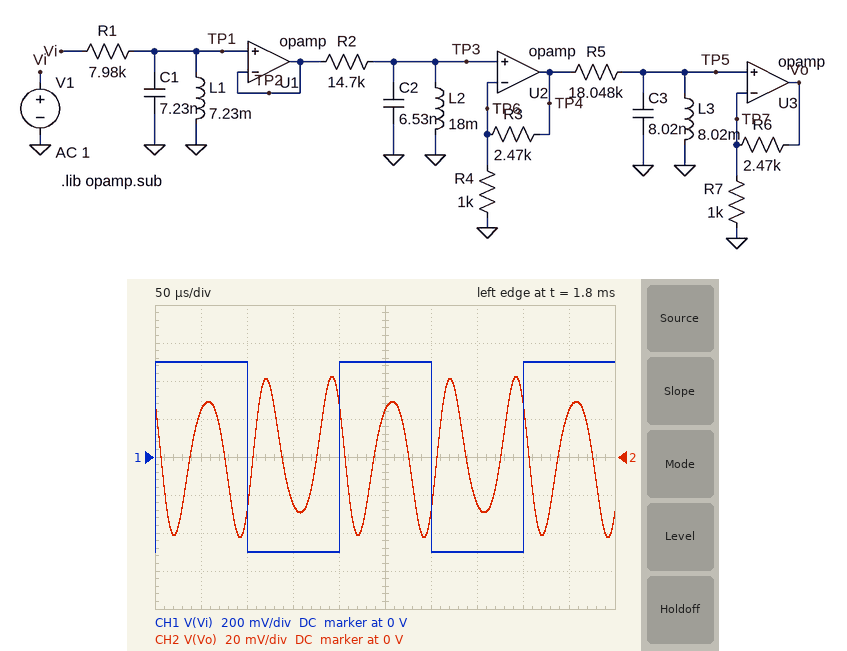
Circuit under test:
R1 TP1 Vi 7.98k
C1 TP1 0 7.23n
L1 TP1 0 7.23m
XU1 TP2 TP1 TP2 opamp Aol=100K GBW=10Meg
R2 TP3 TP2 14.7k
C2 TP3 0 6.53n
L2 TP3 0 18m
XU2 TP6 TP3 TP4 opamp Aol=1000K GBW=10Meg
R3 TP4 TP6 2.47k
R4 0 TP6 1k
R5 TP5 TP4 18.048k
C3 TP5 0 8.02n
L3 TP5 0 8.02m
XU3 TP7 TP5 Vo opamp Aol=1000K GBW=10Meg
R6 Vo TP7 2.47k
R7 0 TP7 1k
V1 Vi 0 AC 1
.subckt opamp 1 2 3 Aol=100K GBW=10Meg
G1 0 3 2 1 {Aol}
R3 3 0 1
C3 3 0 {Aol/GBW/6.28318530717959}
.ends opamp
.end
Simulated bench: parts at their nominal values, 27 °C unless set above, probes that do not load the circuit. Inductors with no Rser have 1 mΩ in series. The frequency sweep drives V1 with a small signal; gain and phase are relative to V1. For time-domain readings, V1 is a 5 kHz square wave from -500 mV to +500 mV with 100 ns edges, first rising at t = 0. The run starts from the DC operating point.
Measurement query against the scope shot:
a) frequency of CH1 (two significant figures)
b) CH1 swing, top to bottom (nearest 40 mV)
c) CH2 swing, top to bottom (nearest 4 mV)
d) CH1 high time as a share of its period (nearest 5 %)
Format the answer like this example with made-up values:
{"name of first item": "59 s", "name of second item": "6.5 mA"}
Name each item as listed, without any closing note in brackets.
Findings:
{"frequency of CH1": "5.0 kHz", "CH1 swing, top to bottom": "1.00 V", "CH2 swing, top to bottom": "84 mV", "CH1 high time as a share of its period": "50 %"}
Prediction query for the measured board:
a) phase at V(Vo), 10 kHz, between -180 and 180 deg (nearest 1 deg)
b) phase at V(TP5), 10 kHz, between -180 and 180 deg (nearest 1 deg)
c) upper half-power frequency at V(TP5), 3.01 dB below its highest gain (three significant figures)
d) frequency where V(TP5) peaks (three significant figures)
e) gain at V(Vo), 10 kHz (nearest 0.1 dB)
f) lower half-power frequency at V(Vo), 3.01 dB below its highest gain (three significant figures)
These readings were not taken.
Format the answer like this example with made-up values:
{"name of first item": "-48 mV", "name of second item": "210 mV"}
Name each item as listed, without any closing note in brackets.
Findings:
{"phase at V(Vo), 10 kHz, between -180 and 180 deg": "-105 deg", "phase at V(TP5), 10 kHz, between -180 and 180 deg": "-105 deg", "upper half-power frequency at V(TP5), 3.01 dB below its highest gain": "20.6 kHz", "frequency where V(TP5) peaks": "19.9 kHz", "gain at V(Vo), 10 kHz": "-46.8 dB", "lower half-power frequency at V(Vo), 3.01 dB below its highest gain": "19.4 kHz"}
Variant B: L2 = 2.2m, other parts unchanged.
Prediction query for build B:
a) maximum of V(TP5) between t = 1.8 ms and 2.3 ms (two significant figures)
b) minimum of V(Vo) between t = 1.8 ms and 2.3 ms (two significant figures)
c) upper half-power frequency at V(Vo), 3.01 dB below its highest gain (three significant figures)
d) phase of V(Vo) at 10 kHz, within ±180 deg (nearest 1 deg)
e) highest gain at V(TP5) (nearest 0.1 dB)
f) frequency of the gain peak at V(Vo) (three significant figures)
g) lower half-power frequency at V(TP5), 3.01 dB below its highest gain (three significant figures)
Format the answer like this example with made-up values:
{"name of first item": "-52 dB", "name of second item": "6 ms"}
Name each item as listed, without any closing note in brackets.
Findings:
{"maximum of V(TP5) between t = 1.8 ms and 2.3 ms": "1.1 mV", "minimum of V(Vo) between t = 1.8 ms and 2.3 ms": "-3.7 mV", "upper half-power frequency at V(Vo), 3.01 dB below its highest gain": "21.1 kHz", "phase of V(Vo) at 10 kHz, within ±180 deg": "-97 deg", "highest gain at V(TP5)": "-27.1 dB", "frequency of the gain peak at V(Vo)": "20.0 kHz", "lower half-power frequency at V(TP5), 3.01 dB below its highest gain": "19.5 kHz"}
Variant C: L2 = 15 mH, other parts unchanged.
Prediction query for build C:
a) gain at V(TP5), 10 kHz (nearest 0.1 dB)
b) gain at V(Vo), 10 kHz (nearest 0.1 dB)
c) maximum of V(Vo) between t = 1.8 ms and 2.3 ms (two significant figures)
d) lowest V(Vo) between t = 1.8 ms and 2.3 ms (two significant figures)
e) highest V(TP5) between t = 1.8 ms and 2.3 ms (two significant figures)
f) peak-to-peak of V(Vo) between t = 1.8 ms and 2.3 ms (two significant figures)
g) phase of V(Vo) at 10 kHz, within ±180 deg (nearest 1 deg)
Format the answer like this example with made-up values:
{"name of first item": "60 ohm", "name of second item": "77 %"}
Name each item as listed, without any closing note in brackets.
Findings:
{"gain at V(TP5), 10 kHz": "-60.3 dB", "gain at V(Vo), 10 kHz": "-49.5 dB", "maximum of V(Vo) between t = 1.8 ms and 2.3 ms": "31 mV", "lowest V(Vo) between t = 1.8 ms and 2.3 ms": "-31 mV", "highest V(TP5) between t = 1.8 ms and 2.3 ms": "8.9 mV", "peak-to-peak of V(Vo) between t = 1.8 ms and 2.3 ms": "62 mV", "phase of V(Vo) at 10 kHz, within ±180 deg": "-103 deg"}
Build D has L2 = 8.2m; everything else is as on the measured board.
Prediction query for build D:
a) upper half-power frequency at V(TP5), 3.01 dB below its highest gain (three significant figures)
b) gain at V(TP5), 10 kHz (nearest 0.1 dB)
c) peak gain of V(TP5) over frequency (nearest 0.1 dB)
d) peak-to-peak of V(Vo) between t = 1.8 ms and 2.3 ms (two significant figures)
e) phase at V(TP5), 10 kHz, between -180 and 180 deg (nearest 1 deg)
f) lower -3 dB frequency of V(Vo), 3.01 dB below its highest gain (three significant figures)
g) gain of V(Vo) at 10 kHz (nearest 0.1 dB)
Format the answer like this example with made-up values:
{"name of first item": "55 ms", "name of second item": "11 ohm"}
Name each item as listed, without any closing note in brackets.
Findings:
{"upper half-power frequency at V(TP5), 3.01 dB below its highest gain": "22.2 kHz", "gain at V(TP5), 10 kHz": "-67.7 dB", "peak gain of V(TP5) over frequency": "0.1 dB", "peak-to-peak of V(Vo) between t = 1.8 ms and 2.3 ms": "49 mV", "phase at V(TP5), 10 kHz, between -180 and 180 deg": "-99 deg", "lower -3 dB frequency of V(Vo), 3.01 dB below its highest gain": "19.9 kHz", "gain of V(Vo) at 10 kHz": "-56.9 dB"}
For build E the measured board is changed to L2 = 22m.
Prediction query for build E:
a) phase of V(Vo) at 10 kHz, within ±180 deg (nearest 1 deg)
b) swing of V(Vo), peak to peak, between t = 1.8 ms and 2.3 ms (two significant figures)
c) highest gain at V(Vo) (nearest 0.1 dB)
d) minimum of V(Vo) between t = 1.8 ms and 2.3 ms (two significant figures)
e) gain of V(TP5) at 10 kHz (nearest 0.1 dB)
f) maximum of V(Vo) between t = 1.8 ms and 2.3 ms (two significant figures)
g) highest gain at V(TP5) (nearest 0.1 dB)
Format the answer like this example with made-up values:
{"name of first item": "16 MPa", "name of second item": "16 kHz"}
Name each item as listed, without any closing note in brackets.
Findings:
{"phase of V(Vo) at 10 kHz, within ±180 deg": "-109 deg", "swing of V(Vo), peak to peak, between t = 1.8 ms and 2.3 ms": "50 mV", "highest gain at V(Vo)": "-0.6 dB", "minimum of V(Vo) between t = 1.8 ms and 2.3 ms": "-25 mV", "gain of V(TP5) at 10 kHz": "-54.1 dB", "maximum of V(Vo) between t = 1.8 ms and 2.3 ms": "25 mV", "highest gain at V(TP5)": "-11.4 dB"}
